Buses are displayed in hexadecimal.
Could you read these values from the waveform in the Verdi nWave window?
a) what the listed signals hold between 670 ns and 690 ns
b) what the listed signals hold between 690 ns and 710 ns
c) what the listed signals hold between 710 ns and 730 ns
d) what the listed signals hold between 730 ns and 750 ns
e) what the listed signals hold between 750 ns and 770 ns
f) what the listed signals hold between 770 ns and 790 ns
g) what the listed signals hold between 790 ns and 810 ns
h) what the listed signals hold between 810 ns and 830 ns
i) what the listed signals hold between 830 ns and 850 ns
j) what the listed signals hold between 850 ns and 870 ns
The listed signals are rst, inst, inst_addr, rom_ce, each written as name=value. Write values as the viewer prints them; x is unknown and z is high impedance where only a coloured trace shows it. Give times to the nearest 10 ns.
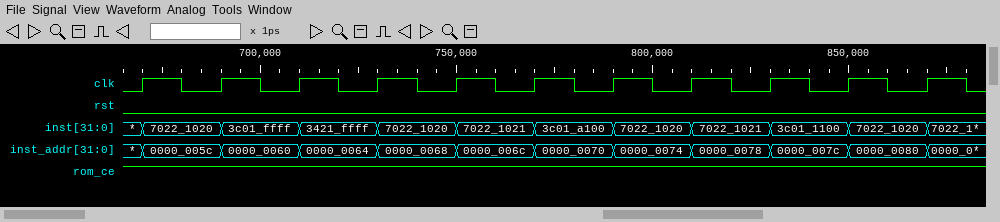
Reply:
rst=0, inst=7022_1020, inst_addr=0000_005c, rom_ce=1
rst=0, inst=3c01_ffff, inst_addr=0000_0060, rom_ce=1
rst=0, inst=3421_ffff, inst_addr=0000_0064, rom_ce=1
rst=0, inst=7022_1020, inst_addr=0000_0068, rom_ce=1
rst=0, inst=7022_1021, inst_addr=0000_006c, rom_ce=1
rst=0, inst=3c01_a100, inst_addr=0000_0070, rom_ce=1
rst=0, inst=7022_1020, inst_addr=0000_0074, rom_ce=1
rst=0, inst=7022_1021, inst_addr=0000_0078, rom_ce=1
rst=0, inst=3c01_1100, inst_addr=0000_007c, rom_ce=1
rst=0, inst=7022_1020, inst_addr=0000_0080, rom_ce=1
